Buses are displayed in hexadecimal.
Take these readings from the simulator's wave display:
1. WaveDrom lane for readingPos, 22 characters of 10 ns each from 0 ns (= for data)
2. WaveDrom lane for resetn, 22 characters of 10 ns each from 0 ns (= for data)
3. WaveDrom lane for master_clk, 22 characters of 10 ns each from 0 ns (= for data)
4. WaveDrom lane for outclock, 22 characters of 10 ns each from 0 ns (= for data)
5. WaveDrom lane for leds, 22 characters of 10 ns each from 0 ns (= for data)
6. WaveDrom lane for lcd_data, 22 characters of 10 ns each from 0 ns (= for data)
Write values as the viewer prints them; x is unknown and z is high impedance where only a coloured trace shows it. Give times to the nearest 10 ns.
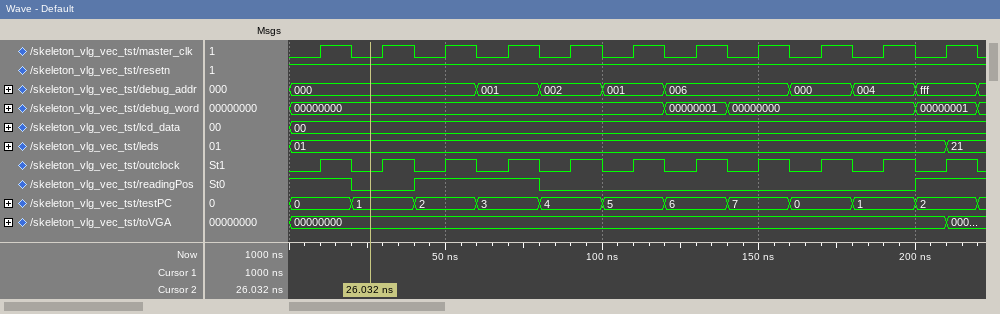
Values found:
{name: 'readingPos', wave: '1.0.1...0...........1.'}
{name: 'resetn', wave: '1.....................'}
{name: 'master_clk', wave: '0101010101010101010101'}
{name: 'outclock', wave: '0101010101010101010101'}
{name: 'leds', wave: '=....................=', data: '01 21'}
{name: 'lcd_data', wave: '=.....................', data: '00'}
